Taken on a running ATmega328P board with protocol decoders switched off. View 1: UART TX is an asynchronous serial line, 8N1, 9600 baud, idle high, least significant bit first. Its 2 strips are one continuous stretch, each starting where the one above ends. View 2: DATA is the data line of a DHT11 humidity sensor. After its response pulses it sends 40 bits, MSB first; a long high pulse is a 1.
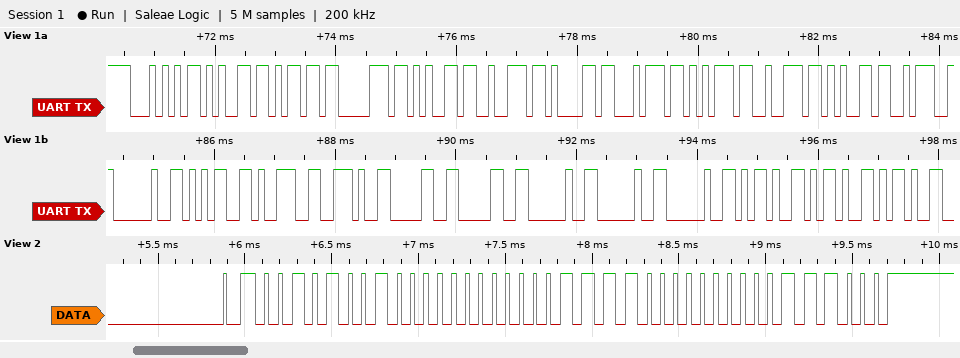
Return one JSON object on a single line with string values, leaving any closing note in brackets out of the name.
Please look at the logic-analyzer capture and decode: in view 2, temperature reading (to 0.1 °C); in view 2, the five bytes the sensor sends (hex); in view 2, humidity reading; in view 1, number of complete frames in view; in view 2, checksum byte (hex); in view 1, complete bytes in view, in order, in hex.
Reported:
{"in view 2, temperature reading": "15.0 °C", "in view 2, the five bytes the sensor sends": "29 00 0F 00 38", "in view 2, humidity reading": "41 %", "in view 1, number of complete frames in view": "24", "in view 2, checksum byte": "0x38", "in view 1, complete bytes in view, in order, in hex": "54 65 6D 70 65 72 61 74 75 72 65 3A 20 35 39 2E 30 30 20 20 20 2D 2D 2D"}
